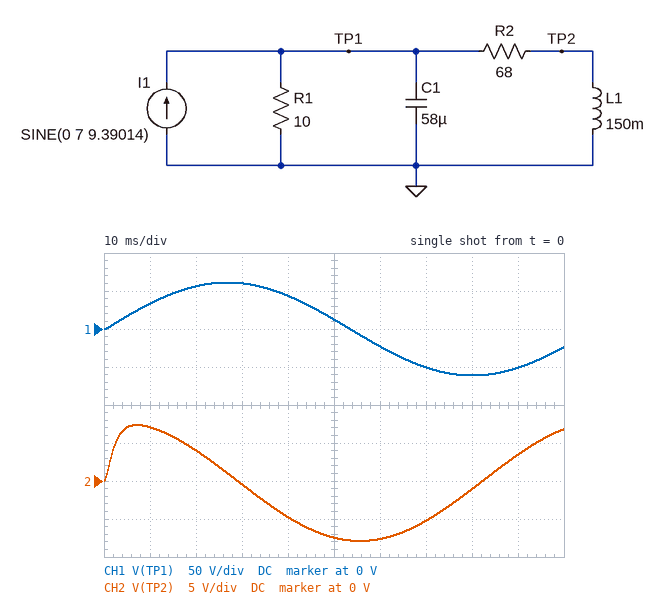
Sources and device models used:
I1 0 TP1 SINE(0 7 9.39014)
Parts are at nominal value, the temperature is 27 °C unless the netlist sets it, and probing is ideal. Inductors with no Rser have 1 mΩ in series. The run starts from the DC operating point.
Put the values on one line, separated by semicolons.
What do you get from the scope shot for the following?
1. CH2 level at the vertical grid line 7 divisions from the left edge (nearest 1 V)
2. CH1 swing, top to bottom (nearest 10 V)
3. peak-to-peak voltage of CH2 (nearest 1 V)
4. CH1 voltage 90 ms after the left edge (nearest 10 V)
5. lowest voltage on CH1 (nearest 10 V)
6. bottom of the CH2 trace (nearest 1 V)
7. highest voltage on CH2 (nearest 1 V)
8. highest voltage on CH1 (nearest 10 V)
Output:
-5 V; 120 V; 15 V; -50 V; -60 V; -8 V; 7 V; 60 V
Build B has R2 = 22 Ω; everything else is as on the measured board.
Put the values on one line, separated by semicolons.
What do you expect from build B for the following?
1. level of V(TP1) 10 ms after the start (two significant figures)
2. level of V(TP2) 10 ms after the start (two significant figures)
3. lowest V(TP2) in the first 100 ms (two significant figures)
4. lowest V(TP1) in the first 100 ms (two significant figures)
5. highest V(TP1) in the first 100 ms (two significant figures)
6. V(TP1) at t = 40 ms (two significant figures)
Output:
31 V; 16 V; -19 V; -50 V; 50 V; 32 V
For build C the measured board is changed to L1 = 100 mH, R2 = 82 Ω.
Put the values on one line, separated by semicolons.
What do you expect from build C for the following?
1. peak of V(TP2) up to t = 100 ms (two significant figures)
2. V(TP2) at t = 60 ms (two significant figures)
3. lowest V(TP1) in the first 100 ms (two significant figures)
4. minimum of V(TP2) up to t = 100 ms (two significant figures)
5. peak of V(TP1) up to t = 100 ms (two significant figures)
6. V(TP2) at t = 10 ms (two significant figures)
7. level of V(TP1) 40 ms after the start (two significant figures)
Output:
4.3 V; -4.3 V; -62 V; -4.5 V; 62 V; 3.9 V; 45 V
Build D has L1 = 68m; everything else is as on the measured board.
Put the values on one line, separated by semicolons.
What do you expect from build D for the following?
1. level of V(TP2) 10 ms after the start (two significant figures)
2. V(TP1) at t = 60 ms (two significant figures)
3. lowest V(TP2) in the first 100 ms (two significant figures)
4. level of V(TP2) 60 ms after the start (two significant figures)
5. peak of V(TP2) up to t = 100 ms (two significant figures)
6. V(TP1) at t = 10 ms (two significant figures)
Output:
3.1 V; -22 V; -3.6 V; -3.4 V; 3.5 V; 33 V
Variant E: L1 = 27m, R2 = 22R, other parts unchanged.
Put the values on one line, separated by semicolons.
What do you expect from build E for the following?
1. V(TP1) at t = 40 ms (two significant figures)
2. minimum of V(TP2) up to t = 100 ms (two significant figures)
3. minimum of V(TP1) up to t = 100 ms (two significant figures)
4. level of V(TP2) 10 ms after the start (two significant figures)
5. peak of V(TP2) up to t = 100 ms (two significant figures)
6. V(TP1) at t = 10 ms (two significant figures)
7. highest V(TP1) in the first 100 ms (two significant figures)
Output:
34 V; -3.5 V; -48 V; 3.0 V; 3.4 V; 27 V; 48 V
